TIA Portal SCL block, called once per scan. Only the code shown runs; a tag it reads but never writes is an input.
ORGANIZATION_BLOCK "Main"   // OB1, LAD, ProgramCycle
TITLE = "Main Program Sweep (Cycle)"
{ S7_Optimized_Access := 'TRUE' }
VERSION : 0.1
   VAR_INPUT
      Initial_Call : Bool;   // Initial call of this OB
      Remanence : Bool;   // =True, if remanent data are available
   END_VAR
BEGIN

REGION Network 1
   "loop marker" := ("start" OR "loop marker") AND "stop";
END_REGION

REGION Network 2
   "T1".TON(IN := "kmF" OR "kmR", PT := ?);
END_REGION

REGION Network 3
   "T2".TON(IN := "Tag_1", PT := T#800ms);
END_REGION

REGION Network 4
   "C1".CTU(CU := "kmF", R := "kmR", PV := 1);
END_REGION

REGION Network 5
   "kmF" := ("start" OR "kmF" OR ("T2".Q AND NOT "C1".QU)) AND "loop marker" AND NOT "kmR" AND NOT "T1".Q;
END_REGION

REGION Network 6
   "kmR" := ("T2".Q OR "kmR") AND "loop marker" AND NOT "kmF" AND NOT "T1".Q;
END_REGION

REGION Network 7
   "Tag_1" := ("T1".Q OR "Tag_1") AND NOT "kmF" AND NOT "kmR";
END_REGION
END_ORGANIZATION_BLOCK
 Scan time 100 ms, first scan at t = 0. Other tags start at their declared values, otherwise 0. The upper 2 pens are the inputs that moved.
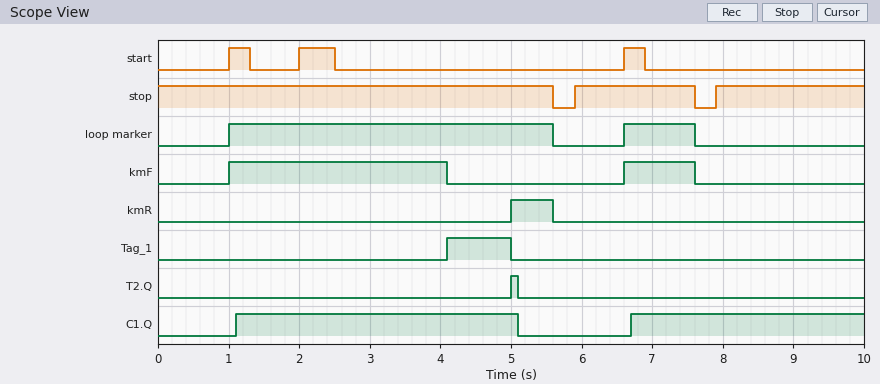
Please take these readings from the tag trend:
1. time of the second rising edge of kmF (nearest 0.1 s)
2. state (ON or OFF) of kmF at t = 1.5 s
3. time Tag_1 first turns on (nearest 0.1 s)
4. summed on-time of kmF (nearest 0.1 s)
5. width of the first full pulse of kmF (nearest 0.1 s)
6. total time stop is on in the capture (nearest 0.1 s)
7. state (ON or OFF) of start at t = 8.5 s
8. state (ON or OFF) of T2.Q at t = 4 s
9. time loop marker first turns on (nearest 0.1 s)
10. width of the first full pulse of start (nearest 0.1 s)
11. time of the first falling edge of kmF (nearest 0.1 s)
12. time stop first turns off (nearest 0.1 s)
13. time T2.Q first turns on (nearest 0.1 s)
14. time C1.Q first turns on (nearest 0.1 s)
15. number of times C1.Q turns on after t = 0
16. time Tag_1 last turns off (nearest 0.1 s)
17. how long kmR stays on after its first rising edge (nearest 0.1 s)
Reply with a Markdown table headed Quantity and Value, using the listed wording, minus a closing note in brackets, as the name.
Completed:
| Quantity | Value |
|---|---|
| time of the second rising edge of kmF | 6.6 s |
| state (ON or OFF) of kmF at t = 1.5 s | ON |
| time Tag_1 first turns on | 4.1 s |
| summed on-time of kmF | 4.1 s |
| width of the first full pulse of kmF | 3.1 s |
| total time stop is on in the capture | 9.4 s |
| state (ON or OFF) of start at t = 8.5 s | OFF |
| state (ON or OFF) of T2.Q at t = 4 s | OFF |
| time loop marker first turns on | 1.0 s |
| width of the first full pulse of start | 0.3 s |
| time of the first falling edge of kmF | 4.1 s |
| time stop first turns off | 5.6 s |
| time T2.Q first turns on | 5.0 s |
| time C1.Q first turns on | 1.1 s |
| number of times C1.Q turns on after t = 0 | 2 |
| time Tag_1 last turns off | 5.0 s |
| how long kmR stays on after its first rising edge | 0.6 s |
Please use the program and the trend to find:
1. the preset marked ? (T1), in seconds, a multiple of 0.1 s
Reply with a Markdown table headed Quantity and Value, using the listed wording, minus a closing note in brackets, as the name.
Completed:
| Quantity | Value |
|---|---|
| the preset marked ? (T1), in seconds, a multiple of 0.1 s | 3.0 s |
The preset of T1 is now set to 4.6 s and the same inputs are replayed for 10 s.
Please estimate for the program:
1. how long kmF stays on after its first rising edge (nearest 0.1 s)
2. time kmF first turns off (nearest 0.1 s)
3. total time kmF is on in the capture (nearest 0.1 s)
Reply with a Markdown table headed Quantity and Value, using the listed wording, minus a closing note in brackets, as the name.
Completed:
| Quantity | Value |
|---|---|
| how long kmF stays on after its first rising edge | 4.6 s |
| time kmF first turns off | 5.6 s |
| total time kmF is on in the capture | 5.6 s |
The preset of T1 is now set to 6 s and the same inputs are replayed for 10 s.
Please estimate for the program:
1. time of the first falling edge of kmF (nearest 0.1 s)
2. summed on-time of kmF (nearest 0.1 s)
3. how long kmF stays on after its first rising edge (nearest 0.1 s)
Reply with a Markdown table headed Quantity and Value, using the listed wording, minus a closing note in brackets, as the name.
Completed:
| Quantity | Value |
|---|---|
| time of the first falling edge of kmF | 5.6 s |
| summed on-time of kmF | 5.6 s |
| how long kmF stays on after its first rising edge | 4.6 s |
